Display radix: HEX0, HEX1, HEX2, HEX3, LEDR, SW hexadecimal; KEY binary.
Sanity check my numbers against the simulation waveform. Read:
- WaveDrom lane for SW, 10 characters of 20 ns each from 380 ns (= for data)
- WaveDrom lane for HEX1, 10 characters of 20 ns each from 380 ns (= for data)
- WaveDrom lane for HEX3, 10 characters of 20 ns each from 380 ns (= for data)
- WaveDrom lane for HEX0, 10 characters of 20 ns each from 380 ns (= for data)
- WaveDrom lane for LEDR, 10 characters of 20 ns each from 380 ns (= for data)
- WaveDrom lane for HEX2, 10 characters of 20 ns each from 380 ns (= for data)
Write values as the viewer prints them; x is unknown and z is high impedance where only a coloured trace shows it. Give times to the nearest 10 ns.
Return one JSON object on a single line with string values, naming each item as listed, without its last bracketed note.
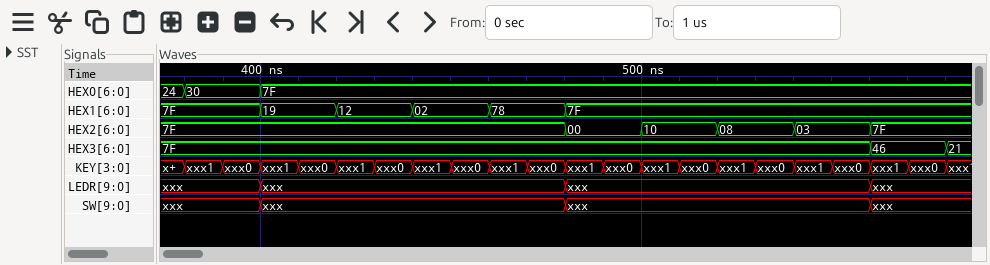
{"WaveDrom lane for SW, 10 characters of 20 ns each from 380 ns": "{name: 'SW', wave: '==...=...=', data: 'xxx xxx xxx xxx'}", "WaveDrom lane for HEX1, 10 characters of 20 ns each from 380 ns": "{name: 'HEX1', wave: '======....', data: '7F 19 12 02 78 7F'}", "WaveDrom lane for HEX3, 10 characters of 20 ns each from 380 ns": "{name: 'HEX3', wave: '=........=', data: '7F 46'}", "WaveDrom lane for HEX0, 10 characters of 20 ns each from 380 ns": "{name: 'HEX0', wave: '==........', data: '30 7F'}", "WaveDrom lane for LEDR, 10 characters of 20 ns each from 380 ns": "{name: 'LEDR', wave: '==...=...=', data: 'xxx xxx xxx xxx'}", "WaveDrom lane for HEX2, 10 characters of 20 ns each from 380 ns": "{name: 'HEX2', wave: '=....=====', data: '7F 00 10 08 03 7F'}"}
